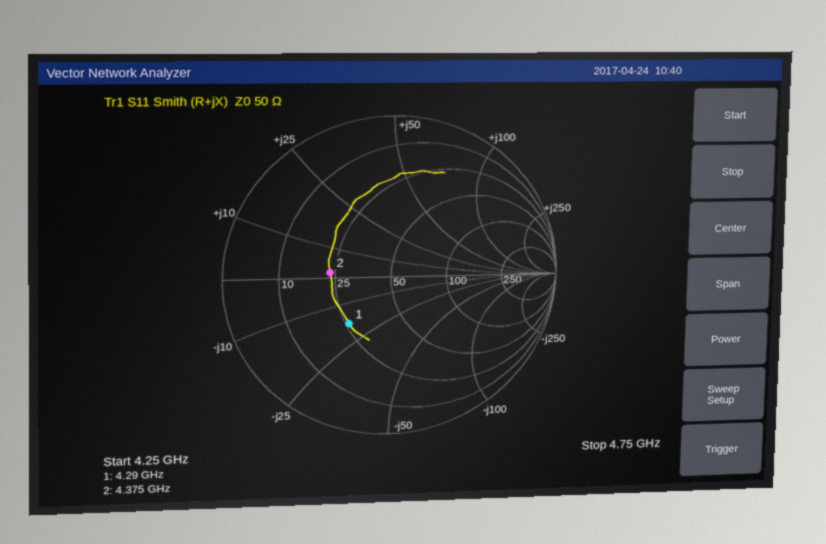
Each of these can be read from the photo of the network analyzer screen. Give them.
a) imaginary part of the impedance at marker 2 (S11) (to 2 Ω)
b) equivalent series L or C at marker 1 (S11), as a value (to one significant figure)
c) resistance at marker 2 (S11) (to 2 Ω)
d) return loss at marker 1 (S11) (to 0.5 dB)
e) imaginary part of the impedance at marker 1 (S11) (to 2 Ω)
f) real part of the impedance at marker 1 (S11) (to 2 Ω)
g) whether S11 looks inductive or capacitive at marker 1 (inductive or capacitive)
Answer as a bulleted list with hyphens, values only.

- +2 Ω
- 2 pF
- 24 Ω
- 8.5 dB
- -18 Ω
- 26 Ω
- capacitive
